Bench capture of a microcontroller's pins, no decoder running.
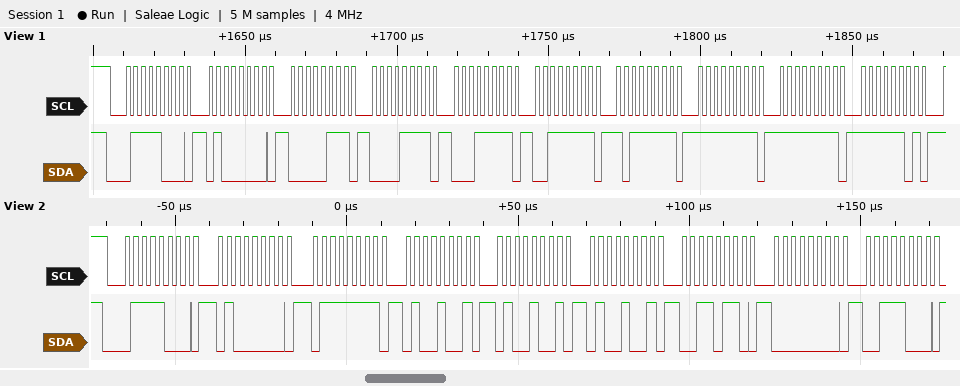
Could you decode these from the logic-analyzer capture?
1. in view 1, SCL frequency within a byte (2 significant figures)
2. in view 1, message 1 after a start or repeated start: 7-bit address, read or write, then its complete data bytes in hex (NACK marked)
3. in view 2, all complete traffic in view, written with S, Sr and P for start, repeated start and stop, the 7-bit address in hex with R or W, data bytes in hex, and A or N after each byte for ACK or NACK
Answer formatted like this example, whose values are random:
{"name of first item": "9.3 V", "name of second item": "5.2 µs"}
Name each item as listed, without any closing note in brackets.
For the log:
{"in view 1, SCL frequency within a byte": "400 kHz", "in view 1, message 1 after a start or repeated start: 7-bit address, read or write, then its complete data bytes in hex": "0x3C write: 40 07 0F 1F 3F BF FF FF FD", "in view 2, all complete traffic in view, written with S, Sr and P for start, repeated start and stop, the 7-bit address in hex with R or W, data bytes in hex, and A or N after each byte for ACK or NACK": "S 3CW A 40 A 7F A 49 A 49 A 49 A 36 A 00 A 38 A"}
